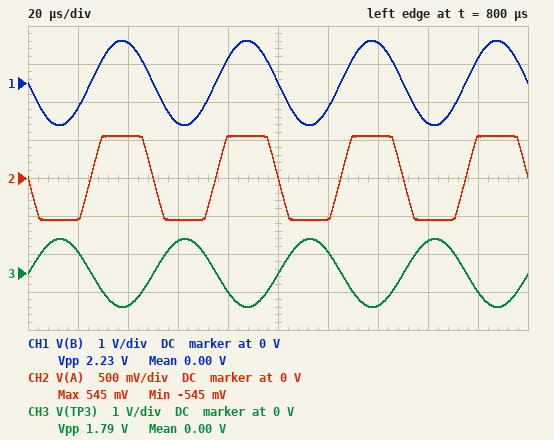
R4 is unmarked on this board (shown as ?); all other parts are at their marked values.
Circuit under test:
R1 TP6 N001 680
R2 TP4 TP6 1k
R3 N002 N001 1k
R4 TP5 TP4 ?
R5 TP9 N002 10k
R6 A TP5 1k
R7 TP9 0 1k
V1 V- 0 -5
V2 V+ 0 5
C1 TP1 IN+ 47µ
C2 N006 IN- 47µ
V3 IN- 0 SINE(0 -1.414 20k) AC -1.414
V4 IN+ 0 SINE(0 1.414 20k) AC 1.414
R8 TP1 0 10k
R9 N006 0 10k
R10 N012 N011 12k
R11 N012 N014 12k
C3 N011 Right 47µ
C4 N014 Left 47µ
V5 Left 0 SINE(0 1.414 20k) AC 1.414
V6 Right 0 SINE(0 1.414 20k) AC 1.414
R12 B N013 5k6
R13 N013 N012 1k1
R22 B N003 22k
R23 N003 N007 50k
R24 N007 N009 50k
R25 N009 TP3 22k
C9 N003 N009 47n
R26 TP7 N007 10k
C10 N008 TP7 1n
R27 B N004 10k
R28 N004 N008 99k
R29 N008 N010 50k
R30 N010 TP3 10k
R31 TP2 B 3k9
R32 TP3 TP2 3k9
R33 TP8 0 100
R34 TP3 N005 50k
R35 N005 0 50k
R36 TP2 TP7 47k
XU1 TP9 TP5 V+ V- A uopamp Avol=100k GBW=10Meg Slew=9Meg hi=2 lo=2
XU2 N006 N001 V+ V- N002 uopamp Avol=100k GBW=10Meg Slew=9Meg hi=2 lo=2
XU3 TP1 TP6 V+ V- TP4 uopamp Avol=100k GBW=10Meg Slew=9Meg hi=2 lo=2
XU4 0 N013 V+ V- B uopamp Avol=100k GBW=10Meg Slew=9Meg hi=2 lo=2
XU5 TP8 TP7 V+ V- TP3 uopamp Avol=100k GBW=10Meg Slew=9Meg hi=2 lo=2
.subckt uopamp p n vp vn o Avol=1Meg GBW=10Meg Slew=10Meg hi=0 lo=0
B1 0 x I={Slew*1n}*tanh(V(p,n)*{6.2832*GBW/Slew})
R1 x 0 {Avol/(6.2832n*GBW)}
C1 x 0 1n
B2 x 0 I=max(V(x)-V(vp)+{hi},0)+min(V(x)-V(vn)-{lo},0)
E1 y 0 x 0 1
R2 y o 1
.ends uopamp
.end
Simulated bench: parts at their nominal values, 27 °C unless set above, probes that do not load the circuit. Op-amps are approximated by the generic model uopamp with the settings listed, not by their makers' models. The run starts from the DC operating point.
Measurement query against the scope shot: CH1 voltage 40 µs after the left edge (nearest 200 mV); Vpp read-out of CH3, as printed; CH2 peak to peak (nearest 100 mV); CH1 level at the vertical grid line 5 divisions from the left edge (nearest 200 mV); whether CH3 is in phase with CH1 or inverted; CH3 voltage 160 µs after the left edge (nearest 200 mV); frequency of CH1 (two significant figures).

1.0 V
1.79 V
1.1 V
0 V
inverted
800 mV
20 kHz
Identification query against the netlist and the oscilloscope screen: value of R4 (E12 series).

12 kΩ
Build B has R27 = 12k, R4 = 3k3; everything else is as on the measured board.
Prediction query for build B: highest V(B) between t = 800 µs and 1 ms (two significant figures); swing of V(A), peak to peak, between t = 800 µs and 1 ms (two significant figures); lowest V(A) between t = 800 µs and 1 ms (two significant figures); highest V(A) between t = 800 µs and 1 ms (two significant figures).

1.1 V
2.5 V
-1.3 V
1.3 V
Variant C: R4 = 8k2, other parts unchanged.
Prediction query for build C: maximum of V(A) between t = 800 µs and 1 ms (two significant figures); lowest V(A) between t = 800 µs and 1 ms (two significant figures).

670 mV
-670 mV
